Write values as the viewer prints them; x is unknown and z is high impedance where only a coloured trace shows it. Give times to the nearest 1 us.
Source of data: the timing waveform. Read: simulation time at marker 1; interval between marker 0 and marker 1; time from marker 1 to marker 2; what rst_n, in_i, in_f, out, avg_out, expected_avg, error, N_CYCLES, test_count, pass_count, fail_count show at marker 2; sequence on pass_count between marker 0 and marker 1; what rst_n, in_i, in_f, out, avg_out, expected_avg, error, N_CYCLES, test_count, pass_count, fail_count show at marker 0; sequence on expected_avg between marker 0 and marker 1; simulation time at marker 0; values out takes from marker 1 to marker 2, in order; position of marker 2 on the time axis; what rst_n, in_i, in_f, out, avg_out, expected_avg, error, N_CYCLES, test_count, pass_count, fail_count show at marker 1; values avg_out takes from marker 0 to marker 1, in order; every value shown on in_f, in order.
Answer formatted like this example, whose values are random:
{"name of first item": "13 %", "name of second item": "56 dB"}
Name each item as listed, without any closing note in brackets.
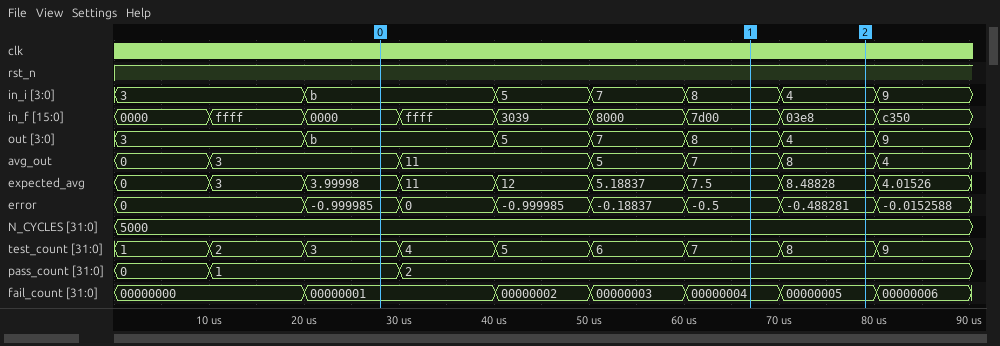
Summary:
{"simulation time at marker 1": "67 us", "interval between marker 0 and marker 1": "39 us", "time from marker 1 to marker 2": "12 us", "what rst_n, in_i, in_f, out, avg_out, expected_avg, error, N_CYCLES, test_count, pass_count, fail_count show at marker 2": "rst_n=1, in_i=4, in_f=03e8, out=4, avg_out=8, expected_avg=8.48828, error=-0.488281, N_CYCLES=5000, test_count=8, pass_count=2, fail_count=00000005", "sequence on pass_count between marker 0 and marker 1": "1, 2", "what rst_n, in_i, in_f, out, avg_out, expected_avg, error, N_CYCLES, test_count, pass_count, fail_count show at marker 0": "rst_n=1, in_i=b, in_f=0000, out=b, avg_out=3, expected_avg=3.99998, error=-0.999985, N_CYCLES=5000, test_count=3, pass_count=1, fail_count=00000001", "sequence on expected_avg between marker 0 and marker 1": "3.99998, 11, 12, 5.18837, 7.5", "simulation time at marker 0": "28 us", "values out takes from marker 1 to marker 2, in order": "8, 4", "position of marker 2 on the time axis": "79 us", "what rst_n, in_i, in_f, out, avg_out, expected_avg, error, N_CYCLES, test_count, pass_count, fail_count show at marker 1": "rst_n=1, in_i=8, in_f=7d00, out=8, avg_out=7, expected_avg=7.5, error=-0.5, N_CYCLES=5000, test_count=7, pass_count=2, fail_count=00000004", "values avg_out takes from marker 0 to marker 1, in order": "3, 11, 5, 7", "every value shown on in_f, in order": "0000, ffff, 0000, ffff, 3039, 8000, 7d00, 03e8, c350"}
